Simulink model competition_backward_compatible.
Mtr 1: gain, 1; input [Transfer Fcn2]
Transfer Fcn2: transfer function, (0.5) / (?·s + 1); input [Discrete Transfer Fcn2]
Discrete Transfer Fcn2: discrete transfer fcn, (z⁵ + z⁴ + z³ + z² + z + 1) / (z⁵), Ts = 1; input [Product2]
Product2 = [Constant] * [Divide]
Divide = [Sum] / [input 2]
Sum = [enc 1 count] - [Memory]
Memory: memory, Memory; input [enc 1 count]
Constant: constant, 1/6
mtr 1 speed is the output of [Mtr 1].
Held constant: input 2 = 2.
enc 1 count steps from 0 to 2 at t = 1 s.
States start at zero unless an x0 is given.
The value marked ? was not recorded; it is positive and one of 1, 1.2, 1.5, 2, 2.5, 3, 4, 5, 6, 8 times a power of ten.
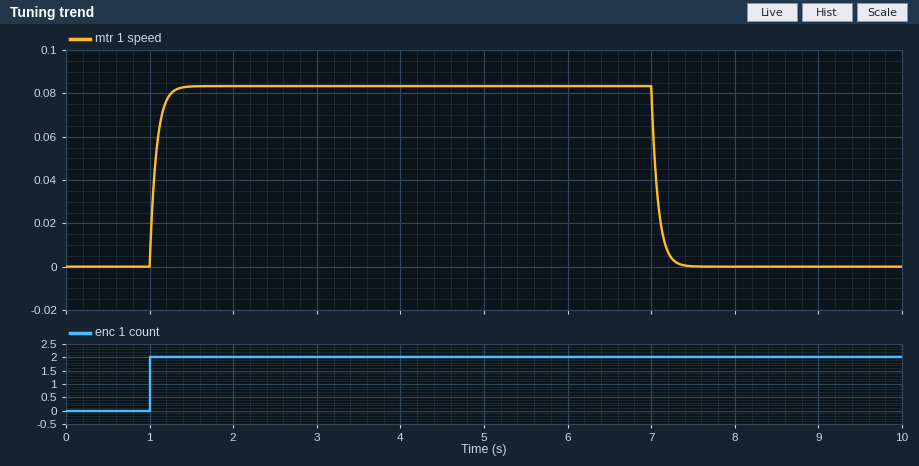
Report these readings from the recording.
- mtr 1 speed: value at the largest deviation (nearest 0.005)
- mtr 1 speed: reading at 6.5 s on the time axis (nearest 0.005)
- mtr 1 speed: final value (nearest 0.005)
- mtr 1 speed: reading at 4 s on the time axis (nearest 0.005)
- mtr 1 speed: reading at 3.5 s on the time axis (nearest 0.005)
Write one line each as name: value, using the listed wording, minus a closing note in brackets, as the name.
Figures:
mtr 1 speed: value at the largest deviation: 0.085
mtr 1 speed: reading at 6.5 s on the time axis: 0.085
mtr 1 speed: final value: 0.000
mtr 1 speed: reading at 4 s on the time axis: 0.085
mtr 1 speed: reading at 3.5 s on the time axis: 0.085
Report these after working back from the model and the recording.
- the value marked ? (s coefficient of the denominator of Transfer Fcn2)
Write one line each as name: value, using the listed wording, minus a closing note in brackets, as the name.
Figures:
the value marked ?: 0.08
